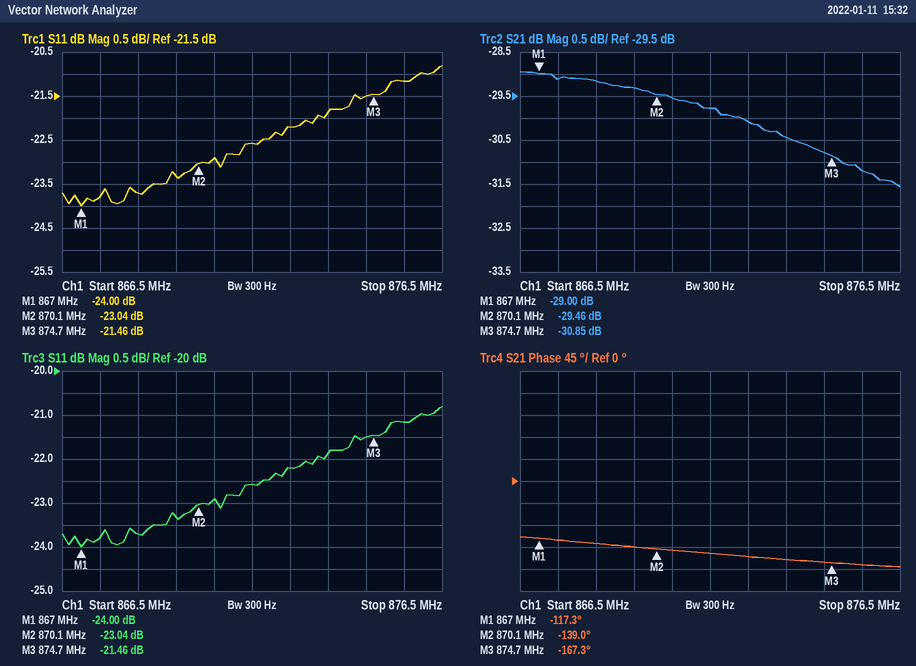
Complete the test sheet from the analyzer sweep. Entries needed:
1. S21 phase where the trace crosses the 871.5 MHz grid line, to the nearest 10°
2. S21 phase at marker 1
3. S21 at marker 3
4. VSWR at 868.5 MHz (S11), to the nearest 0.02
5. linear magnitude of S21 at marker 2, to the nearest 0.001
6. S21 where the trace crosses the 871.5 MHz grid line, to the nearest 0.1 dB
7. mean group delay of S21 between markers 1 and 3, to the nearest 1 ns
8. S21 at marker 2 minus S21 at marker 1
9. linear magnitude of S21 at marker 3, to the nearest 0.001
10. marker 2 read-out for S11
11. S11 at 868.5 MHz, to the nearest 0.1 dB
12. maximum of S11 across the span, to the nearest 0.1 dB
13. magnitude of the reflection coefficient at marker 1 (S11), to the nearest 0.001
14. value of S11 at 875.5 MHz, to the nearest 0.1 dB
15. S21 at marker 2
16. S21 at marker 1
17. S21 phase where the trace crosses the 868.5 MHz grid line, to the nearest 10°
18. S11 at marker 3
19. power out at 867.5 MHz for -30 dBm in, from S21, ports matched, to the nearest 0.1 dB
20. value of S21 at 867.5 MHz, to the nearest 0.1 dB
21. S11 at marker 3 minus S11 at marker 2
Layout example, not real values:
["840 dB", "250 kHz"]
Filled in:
["-150°", "-117.3°", "-30.85 dB", "1.14", "0.034", "-29.8 dB", "18 ns", "-0.46 dB", "0.029", "-23.04 dB", "-23.7 dB", "-20.8 dB", "0.063", "-21.2 dB", "-29.46 dB", "-29.00 dB", "-130°", "-21.46 dB", "-59.1 dBm", "-29.1 dB", "1.58 dB"]
